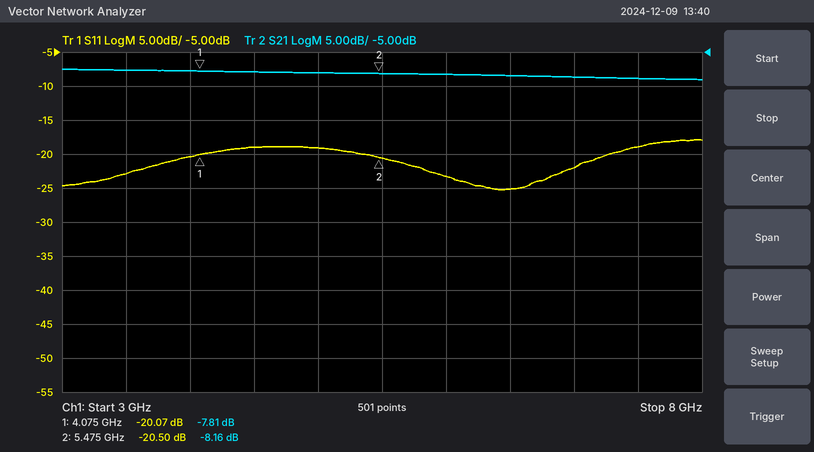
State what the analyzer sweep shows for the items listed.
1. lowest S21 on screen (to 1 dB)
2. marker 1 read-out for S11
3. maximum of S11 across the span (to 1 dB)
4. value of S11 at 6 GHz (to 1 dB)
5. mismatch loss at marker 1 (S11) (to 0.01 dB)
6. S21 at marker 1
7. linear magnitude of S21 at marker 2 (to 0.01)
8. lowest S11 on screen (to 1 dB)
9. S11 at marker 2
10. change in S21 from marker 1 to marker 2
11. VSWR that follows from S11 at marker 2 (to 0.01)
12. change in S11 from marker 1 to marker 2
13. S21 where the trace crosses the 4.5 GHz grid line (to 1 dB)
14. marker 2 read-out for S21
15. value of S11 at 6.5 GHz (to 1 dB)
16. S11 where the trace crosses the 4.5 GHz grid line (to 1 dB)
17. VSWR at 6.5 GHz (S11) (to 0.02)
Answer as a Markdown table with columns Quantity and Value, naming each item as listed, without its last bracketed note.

| Quantity | Value |
|---|---|
| lowest S21 on screen | -9 dB |
| marker 1 read-out for S11 | -20.07 dB |
| maximum of S11 across the span | -18 dB |
| value of S11 at 6 GHz | -23 dB |
| mismatch loss at marker 1 (S11) | 0.04 dB |
| S21 at marker 1 | -7.81 dB |
| linear magnitude of S21 at marker 2 | 0.39 |
| lowest S11 on screen | -25 dB |
| S11 at marker 2 | -20.50 dB |
| change in S21 from marker 1 to marker 2 | -0.35 dB |
| VSWR that follows from S11 at marker 2 | 1.21 |
| change in S11 from marker 1 to marker 2 | -0.43 dB |
| S21 where the trace crosses the 4.5 GHz grid line | -8 dB |
| marker 2 read-out for S21 | -8.16 dB |
| value of S11 at 6.5 GHz | -25 dB |
| S11 where the trace crosses the 4.5 GHz grid line | -19 dB |
| VSWR at 6.5 GHz (S11) | 1.12 |
